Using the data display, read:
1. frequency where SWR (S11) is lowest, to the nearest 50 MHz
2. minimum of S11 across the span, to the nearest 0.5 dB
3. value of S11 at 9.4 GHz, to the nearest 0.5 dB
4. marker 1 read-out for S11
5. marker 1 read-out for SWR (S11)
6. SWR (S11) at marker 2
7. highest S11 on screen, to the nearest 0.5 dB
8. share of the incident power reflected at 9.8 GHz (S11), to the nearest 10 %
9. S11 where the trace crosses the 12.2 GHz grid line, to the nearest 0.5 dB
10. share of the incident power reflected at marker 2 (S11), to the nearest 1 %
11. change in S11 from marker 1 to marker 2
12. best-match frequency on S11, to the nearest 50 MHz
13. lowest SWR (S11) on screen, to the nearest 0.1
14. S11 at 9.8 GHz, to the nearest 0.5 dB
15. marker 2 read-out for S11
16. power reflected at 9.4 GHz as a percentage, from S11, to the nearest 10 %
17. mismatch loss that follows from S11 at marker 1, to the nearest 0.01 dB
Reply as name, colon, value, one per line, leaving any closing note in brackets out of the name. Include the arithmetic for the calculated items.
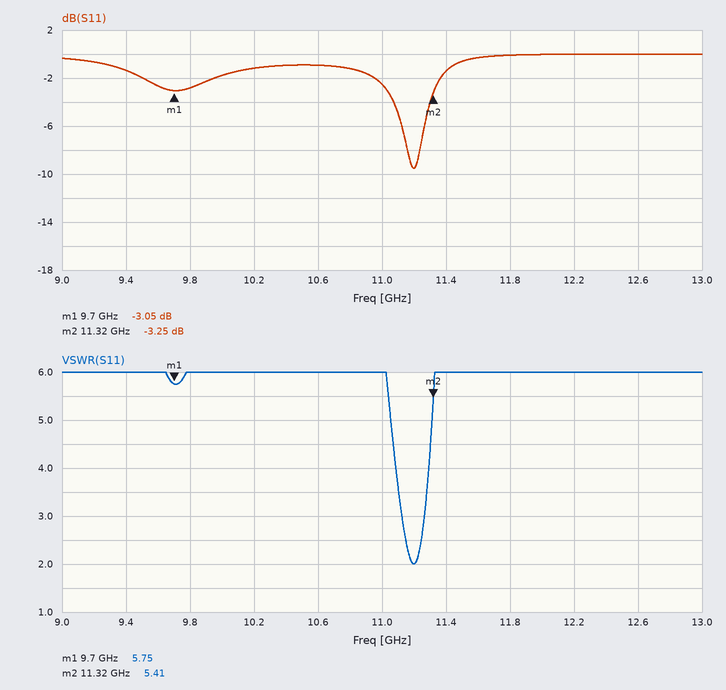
frequency where SWR (S11) is lowest, to the nearest 50 MHz: 11.20 GHz
minimum of S11 across the span, to the nearest 0.5 dB: -9.5 dB
value of S11 at 9.4 GHz, to the nearest 0.5 dB: -1.5 dB
marker 1 read-out for S11: -3.05 dB
marker 1 read-out for SWR: 5.75
SWR (S11) at marker 2: 5.41
highest S11 on screen, to the nearest 0.5 dB: 0.0 dB
share of the incident power reflected at 9.8 GHz (S11), to the nearest 10 %: 10^(-3/10) ≈ 50 %
S11 where the trace crosses the 12.2 GHz grid line, to the nearest 0.5 dB: 0.0 dB
share of the incident power reflected at marker 2 (S11), to the nearest 1 %: 10^(-3.25/10) ≈ 47 %
change in S11 from marker 1 to marker 2: -3.25 − (-3.05) = -0.20 dB
best-match frequency on S11, to the nearest 50 MHz: 11.20 GHz
lowest SWR (S11) on screen, to the nearest 0.1: 2.0
S11 at 9.8 GHz, to the nearest 0.5 dB: -3.0 dB
marker 2 read-out for S11: -3.25 dB
power reflected at 9.4 GHz as a percentage, from S11, to the nearest 10 %: 10^(-1.5/10) ≈ 70.8 %, so 70 % to the nearest 10 %
mismatch loss that follows from S11 at marker 1, to the nearest 0.01 dB: −10 log10(1 − 10^(-3.05/10)) ≈ 2.97 dB
